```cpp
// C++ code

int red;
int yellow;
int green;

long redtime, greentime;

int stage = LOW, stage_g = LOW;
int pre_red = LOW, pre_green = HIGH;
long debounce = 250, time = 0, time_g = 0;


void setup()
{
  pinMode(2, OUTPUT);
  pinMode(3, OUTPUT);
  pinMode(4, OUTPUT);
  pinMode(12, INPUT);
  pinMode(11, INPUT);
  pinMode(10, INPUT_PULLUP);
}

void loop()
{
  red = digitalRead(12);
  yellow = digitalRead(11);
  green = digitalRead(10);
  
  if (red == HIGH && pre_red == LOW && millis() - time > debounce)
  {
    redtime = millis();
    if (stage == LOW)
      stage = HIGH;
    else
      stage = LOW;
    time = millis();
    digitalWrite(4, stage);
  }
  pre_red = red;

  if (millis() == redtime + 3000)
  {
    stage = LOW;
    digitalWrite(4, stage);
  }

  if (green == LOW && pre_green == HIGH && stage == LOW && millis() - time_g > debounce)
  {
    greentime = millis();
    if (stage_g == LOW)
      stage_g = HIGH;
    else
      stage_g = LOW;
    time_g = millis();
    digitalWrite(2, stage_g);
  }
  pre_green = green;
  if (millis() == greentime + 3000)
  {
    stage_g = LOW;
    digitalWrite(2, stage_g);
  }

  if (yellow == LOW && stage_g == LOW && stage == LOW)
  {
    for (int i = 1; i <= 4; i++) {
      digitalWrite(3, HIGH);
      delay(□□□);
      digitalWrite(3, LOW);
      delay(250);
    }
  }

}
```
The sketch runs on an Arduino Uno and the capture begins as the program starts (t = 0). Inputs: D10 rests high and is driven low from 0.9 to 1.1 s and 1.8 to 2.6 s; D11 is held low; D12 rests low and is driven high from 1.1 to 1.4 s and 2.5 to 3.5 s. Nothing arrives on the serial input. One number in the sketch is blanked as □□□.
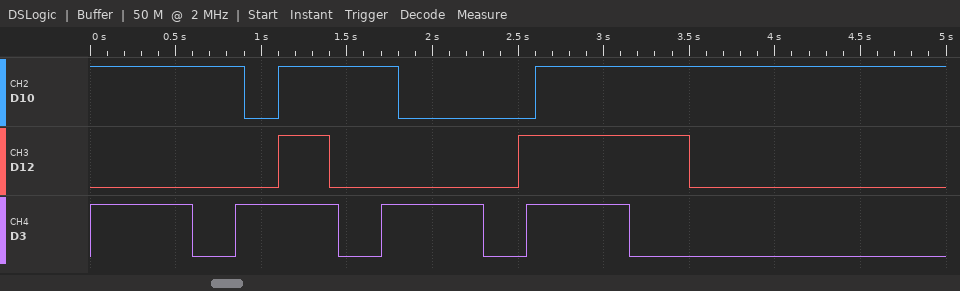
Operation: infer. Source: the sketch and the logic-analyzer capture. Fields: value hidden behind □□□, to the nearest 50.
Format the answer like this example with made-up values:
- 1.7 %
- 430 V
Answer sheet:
- 600
